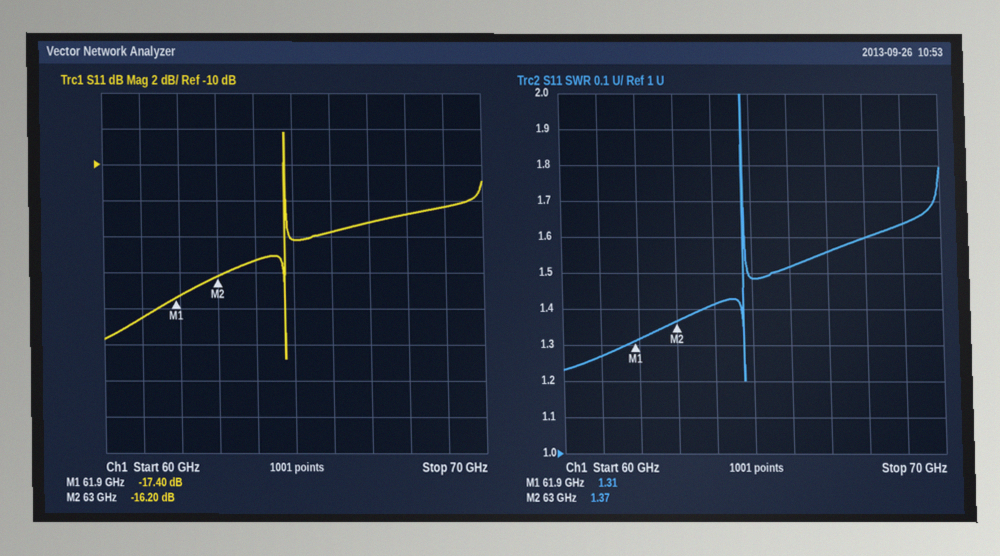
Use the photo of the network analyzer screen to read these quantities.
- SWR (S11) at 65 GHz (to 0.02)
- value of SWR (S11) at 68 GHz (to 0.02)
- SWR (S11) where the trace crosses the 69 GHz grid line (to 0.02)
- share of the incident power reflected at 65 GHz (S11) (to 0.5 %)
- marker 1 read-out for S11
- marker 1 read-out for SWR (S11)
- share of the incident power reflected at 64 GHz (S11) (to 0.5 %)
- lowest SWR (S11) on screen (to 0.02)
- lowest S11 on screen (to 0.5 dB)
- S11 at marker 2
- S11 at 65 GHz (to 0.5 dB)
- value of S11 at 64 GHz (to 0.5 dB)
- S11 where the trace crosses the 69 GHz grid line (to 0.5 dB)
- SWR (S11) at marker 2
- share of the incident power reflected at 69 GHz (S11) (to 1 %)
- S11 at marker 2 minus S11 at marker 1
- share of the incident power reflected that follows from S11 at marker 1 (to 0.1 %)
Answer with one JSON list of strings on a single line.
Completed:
["1.48", "1.60", "1.64", "4.0 %", "-17.40 dB", "1.31", "3.0 %", "1.20", "-21.0 dB", "-16.20 dB", "-14.0 dB", "-15.5 dB", "-12.5 dB", "1.37", "6 %", "1.20 dB", "1.8 %"]
